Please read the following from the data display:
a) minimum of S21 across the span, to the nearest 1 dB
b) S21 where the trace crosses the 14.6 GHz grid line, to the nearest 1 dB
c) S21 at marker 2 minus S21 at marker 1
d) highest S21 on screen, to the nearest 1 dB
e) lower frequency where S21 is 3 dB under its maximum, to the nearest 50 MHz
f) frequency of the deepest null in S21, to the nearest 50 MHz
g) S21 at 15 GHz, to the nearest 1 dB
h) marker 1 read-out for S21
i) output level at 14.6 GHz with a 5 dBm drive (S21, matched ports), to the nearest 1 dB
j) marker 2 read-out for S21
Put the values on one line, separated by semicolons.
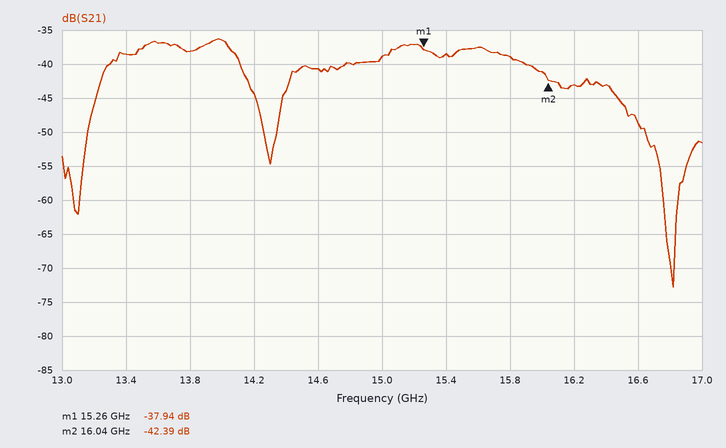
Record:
-73 dB; -41 dB; -4.45 dB; -36 dB; 13.35 GHz; 16.80 GHz; -39 dB; -37.94 dB; -36 dBm; -42.39 dB
